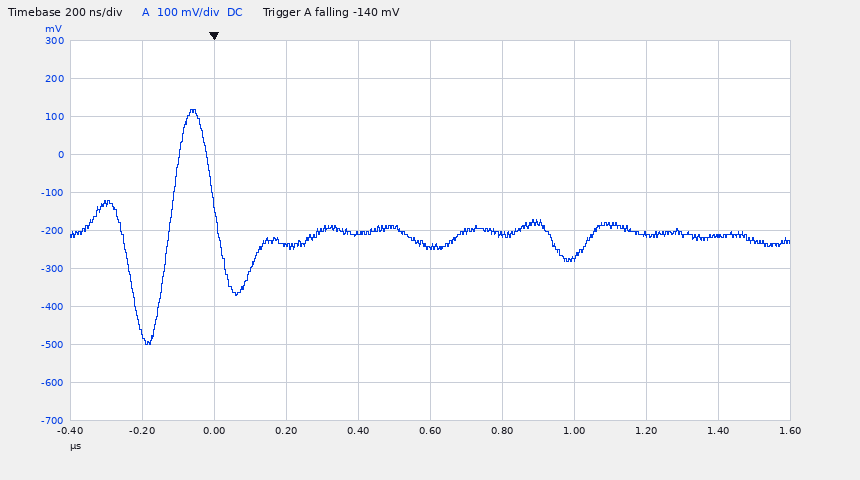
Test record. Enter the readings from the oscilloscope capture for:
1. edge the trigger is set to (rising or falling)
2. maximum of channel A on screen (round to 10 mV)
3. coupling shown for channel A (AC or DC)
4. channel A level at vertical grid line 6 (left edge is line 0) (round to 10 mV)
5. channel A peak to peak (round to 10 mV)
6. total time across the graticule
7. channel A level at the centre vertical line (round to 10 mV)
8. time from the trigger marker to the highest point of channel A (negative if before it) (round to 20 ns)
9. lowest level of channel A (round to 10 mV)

falling
120 mV
DC
-210 mV
620 mV
2 µs
-240 mV
-60 ns
-500 mV
